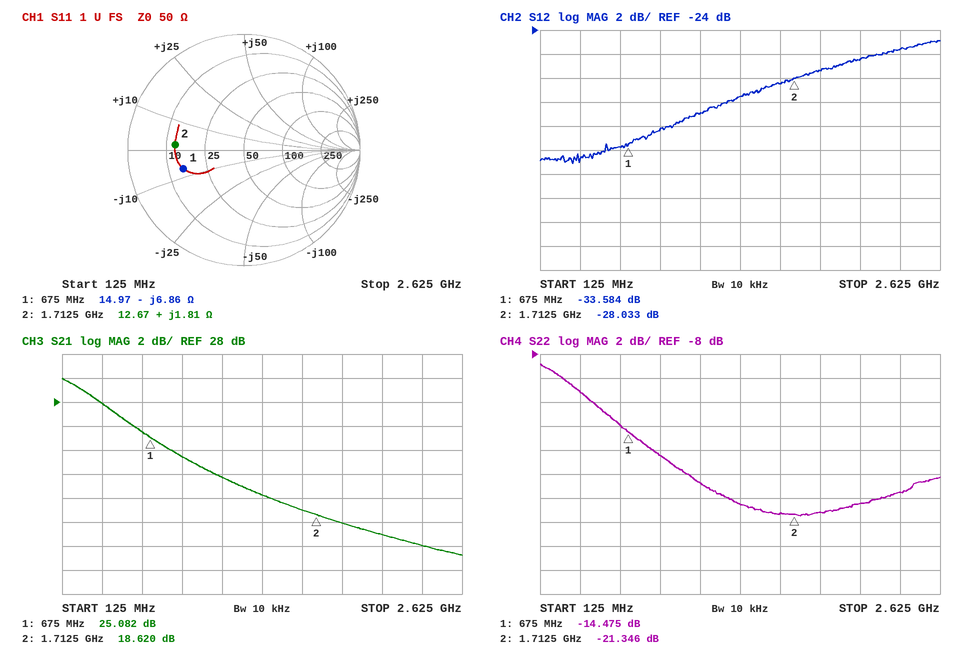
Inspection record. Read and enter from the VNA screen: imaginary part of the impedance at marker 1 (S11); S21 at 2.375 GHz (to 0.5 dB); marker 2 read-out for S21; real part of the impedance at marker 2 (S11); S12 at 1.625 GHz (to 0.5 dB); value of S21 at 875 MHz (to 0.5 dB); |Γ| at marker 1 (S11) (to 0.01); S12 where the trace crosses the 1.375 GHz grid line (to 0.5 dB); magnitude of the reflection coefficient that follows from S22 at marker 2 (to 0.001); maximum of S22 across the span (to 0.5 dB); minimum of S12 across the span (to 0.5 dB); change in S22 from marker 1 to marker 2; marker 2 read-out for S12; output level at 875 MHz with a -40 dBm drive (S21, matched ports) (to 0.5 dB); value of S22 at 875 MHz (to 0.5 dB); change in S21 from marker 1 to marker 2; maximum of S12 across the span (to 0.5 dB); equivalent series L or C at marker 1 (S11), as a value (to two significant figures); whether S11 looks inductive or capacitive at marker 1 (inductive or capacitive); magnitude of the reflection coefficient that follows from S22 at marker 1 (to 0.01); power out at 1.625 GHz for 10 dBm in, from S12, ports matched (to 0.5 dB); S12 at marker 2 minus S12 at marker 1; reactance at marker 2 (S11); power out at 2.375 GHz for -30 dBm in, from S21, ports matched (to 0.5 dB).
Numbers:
-6.86 Ω
16.0 dB
18.620 dB
12.67 Ω
-28.5 dB
23.5 dB
0.55
-29.5 dB
0.086
-9.0 dB
-35.0 dB
-6.871 dB
-28.033 dB
-16.5 dBm
-16.5 dB
-6.462 dB
-25.0 dB
34 pF
capacitive
0.19
-18.5 dBm
5.551 dB
+1.81 Ω
-14.0 dBm
